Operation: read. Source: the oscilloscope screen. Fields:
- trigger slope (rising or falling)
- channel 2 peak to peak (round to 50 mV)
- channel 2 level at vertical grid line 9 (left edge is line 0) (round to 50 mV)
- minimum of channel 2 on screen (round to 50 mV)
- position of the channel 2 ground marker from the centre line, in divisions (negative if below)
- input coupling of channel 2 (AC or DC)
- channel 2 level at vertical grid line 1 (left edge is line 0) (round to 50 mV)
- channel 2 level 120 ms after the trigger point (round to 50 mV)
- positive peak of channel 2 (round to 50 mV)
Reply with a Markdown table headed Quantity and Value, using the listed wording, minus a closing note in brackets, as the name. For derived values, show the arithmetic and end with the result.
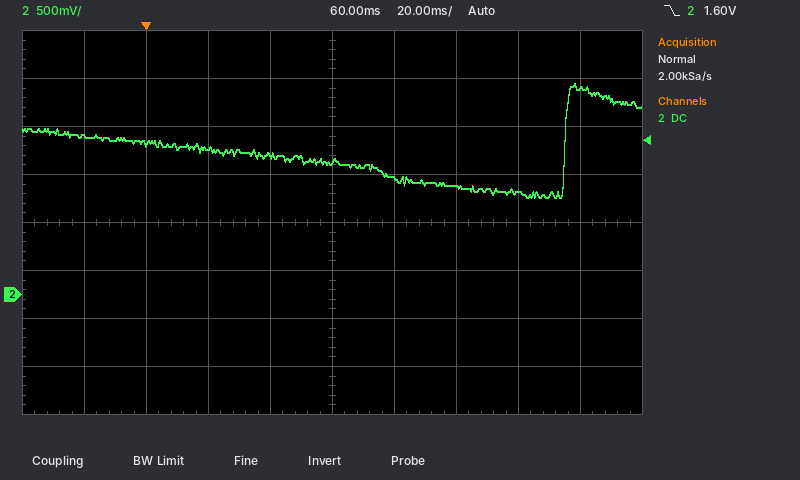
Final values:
| Quantity | Value |
|---|---|
| trigger slope | falling |
| channel 2 peak to peak | 2.20 V − (1.00 V) = 1.20 V |
| channel 2 level at vertical grid line 9 (left edge is line 0) | 2.15 V |
| minimum of channel 2 on screen | 1.00 V |
| position of the channel 2 ground marker from the centre line, in divisions | -1.5 div |
| input coupling of channel 2 | DC |
| channel 2 level at vertical grid line 1 (left edge is line 0) | 1.65 V |
| channel 2 level 120 ms after the trigger point | 1.05 V |
| positive peak of channel 2 | 2.20 V |
